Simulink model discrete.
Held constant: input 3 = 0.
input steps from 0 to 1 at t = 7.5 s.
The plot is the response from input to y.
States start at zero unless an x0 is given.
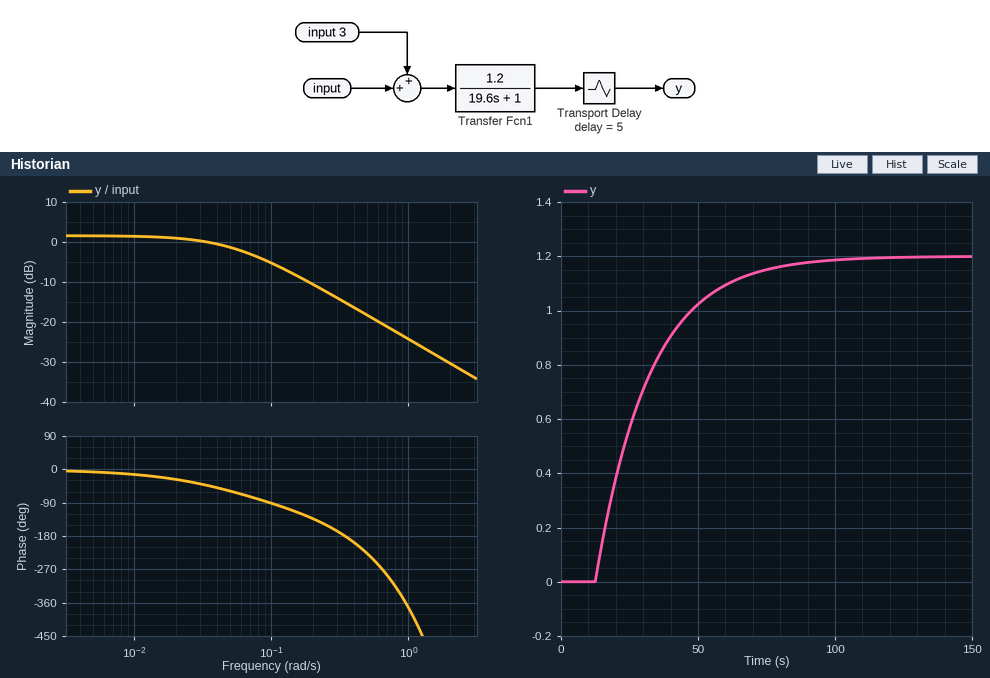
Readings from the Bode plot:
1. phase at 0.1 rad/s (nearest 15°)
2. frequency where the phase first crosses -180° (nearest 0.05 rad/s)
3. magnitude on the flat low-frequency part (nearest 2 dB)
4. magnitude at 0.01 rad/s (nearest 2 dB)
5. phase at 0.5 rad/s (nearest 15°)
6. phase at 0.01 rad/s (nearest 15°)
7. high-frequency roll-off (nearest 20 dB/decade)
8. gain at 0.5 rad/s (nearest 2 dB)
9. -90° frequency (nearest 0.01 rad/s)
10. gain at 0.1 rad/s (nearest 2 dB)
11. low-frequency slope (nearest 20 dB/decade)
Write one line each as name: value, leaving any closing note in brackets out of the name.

phase at 0.1 rad/s: -90°
frequency where the phase first crosses -180°: 0.35 rad/s
magnitude on the flat low-frequency part: 2 dB
magnitude at 0.01 rad/s: 2 dB
phase at 0.5 rad/s: -225°
phase at 0.01 rad/s: -15°
high-frequency roll-off: -20 dB/decade
gain at 0.5 rad/s: -18 dB
-90° frequency: 0.10 rad/s
gain at 0.1 rad/s: -6 dB
low-frequency slope: 0 dB/decade
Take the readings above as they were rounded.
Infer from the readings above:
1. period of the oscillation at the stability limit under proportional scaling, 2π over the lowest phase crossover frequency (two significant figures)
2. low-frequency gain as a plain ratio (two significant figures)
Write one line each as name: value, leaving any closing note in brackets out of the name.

period of the oscillation at the stability limit under proportional scaling, 2π over the lowest phase crossover frequency: 18 s
low-frequency gain as a plain ratio: 1.3
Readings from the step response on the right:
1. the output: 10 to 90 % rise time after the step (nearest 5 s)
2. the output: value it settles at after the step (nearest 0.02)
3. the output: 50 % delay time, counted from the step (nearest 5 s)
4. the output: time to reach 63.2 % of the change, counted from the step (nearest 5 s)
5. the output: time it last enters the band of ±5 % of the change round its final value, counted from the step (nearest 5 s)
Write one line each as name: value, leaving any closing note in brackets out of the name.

the output: 10 to 90 % rise time after the step: 45 s
the output: value it settles at after the step: 1.20
the output: 50 % delay time, counted from the step: 20 s
the output: time to reach 63.2 % of the change, counted from the step: 25 s
the output: time it last enters the band of ±5 % of the change round its final value, counted from the step: 65 s
